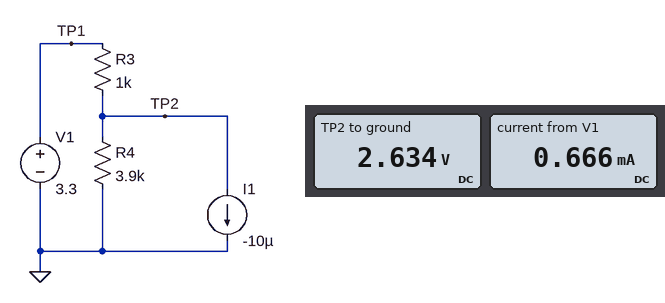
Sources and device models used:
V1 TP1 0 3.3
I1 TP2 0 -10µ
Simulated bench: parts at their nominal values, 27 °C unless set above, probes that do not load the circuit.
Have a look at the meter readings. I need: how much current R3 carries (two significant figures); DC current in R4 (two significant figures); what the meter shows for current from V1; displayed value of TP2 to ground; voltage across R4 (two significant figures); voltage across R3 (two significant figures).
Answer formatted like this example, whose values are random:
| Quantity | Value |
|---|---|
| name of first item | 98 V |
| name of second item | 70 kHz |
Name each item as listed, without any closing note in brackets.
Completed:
| Quantity | Value |
|---|---|
| how much current R3 carries | 670 µA |
| DC current in R4 | 680 µA |
| what the meter shows for current from V1 | 0.666 mA |
| displayed value of TP2 to ground | 2.634 V |
| voltage across R4 | 2.6 V |
| voltage across R3 | 670 mV |
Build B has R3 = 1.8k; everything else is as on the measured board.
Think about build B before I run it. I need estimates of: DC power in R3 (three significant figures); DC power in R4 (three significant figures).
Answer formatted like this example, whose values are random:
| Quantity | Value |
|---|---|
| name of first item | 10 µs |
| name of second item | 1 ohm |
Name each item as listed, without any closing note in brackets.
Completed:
| Quantity | Value |
|---|---|
| DC power in R3 | 589 µW |
| DC power in R4 | 1.32 mW |
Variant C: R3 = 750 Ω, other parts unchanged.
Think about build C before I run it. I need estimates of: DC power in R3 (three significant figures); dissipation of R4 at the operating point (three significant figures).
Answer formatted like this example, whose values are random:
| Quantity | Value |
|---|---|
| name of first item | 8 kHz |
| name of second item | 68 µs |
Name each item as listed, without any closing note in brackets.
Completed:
| Quantity | Value |
|---|---|
| DC power in R3 | 369 µW |
| dissipation of R4 at the operating point | 1.97 mW |
